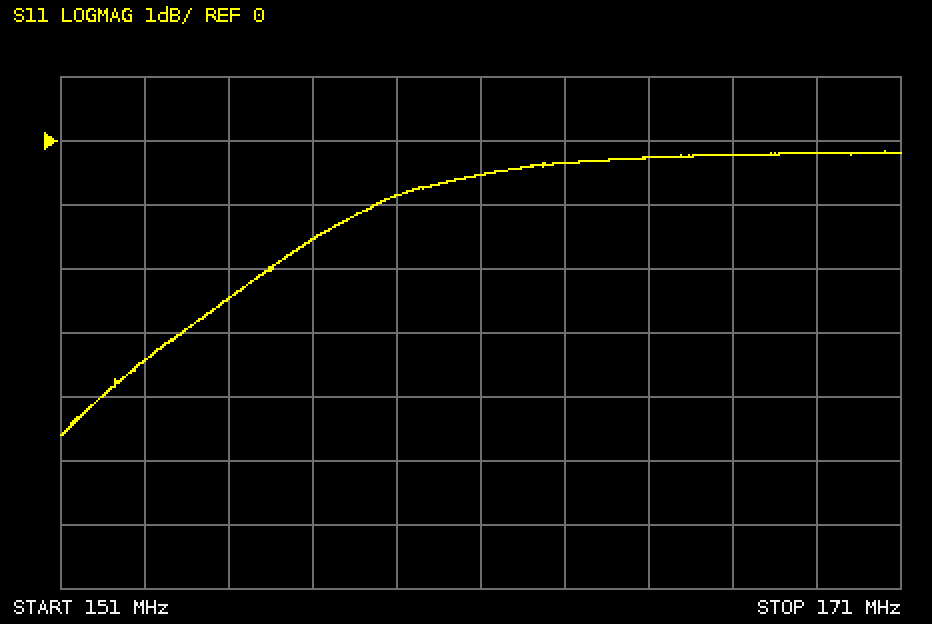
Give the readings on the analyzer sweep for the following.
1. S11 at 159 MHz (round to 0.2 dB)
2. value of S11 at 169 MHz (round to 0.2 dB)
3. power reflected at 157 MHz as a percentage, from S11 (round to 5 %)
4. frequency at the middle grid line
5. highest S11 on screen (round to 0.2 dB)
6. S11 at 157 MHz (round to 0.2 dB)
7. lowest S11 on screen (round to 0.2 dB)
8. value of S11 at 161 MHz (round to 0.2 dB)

-0.8 dB
-0.2 dB
70 %
161 MHz
-0.2 dB
-1.6 dB
-4.6 dB
-0.6 dB
